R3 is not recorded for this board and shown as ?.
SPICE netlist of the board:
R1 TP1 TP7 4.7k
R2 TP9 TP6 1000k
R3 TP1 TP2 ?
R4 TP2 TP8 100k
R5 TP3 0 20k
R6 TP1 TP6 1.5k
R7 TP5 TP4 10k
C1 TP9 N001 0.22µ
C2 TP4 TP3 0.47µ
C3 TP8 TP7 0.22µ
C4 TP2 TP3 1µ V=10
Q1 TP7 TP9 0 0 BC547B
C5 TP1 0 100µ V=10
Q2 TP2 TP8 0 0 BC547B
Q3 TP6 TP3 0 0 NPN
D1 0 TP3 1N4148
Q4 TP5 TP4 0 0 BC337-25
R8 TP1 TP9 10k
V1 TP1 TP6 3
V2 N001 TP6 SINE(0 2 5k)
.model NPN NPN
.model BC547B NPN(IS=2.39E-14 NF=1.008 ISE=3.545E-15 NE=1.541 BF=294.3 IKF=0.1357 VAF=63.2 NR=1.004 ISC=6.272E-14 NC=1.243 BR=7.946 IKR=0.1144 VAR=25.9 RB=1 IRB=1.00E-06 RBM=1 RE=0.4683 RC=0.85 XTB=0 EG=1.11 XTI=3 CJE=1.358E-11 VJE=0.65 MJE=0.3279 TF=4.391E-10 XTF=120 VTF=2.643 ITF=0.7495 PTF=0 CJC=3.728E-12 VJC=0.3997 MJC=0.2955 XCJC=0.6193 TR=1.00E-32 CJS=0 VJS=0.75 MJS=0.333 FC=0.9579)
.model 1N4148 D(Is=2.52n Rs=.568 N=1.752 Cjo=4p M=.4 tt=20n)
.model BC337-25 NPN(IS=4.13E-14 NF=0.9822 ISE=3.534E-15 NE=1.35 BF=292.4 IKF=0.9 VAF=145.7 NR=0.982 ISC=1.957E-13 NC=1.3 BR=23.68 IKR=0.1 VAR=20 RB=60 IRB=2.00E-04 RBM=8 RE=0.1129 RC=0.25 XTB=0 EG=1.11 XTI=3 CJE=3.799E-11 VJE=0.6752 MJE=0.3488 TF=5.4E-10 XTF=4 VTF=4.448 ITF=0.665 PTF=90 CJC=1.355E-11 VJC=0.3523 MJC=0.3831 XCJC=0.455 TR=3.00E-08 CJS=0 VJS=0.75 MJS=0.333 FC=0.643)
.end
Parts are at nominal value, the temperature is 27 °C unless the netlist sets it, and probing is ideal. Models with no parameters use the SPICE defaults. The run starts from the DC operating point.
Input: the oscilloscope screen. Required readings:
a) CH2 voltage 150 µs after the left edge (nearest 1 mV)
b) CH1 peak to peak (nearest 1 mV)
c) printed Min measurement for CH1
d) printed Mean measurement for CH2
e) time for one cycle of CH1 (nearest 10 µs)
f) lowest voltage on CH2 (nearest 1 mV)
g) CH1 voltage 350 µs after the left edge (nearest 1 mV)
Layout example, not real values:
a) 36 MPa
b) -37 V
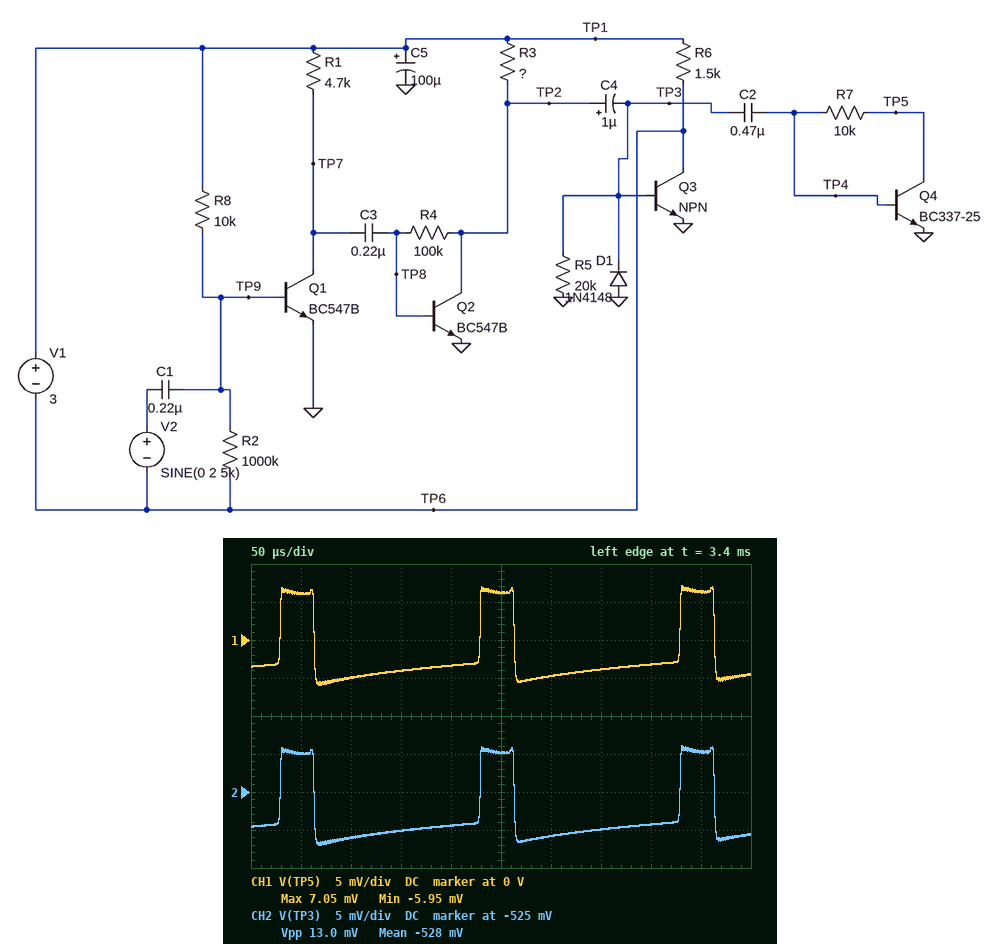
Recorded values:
a) -530 mV
b) 13 mV
c) -5.95 mV
d) -528 mV
e) 200 µs
f) -532 mV
g) -4 mV
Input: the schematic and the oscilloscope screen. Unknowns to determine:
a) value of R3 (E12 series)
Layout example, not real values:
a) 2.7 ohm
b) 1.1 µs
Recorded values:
a) 8.2 kΩ
